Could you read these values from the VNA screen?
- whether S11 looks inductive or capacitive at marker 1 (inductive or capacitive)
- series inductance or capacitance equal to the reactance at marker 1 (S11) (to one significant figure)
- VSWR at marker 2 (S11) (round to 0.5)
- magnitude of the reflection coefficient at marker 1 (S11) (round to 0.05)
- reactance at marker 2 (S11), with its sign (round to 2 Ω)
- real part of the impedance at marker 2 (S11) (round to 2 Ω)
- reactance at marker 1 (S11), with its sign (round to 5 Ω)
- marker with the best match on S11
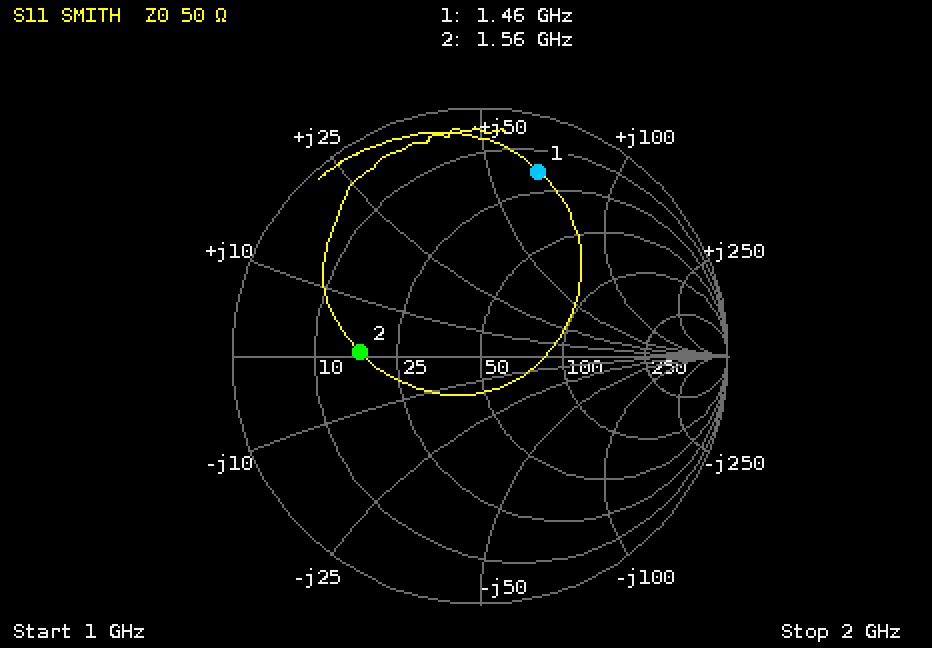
inductive
7 nH
3.0
0.80
0 Ω
18 Ω
+65 Ω
marker 2
